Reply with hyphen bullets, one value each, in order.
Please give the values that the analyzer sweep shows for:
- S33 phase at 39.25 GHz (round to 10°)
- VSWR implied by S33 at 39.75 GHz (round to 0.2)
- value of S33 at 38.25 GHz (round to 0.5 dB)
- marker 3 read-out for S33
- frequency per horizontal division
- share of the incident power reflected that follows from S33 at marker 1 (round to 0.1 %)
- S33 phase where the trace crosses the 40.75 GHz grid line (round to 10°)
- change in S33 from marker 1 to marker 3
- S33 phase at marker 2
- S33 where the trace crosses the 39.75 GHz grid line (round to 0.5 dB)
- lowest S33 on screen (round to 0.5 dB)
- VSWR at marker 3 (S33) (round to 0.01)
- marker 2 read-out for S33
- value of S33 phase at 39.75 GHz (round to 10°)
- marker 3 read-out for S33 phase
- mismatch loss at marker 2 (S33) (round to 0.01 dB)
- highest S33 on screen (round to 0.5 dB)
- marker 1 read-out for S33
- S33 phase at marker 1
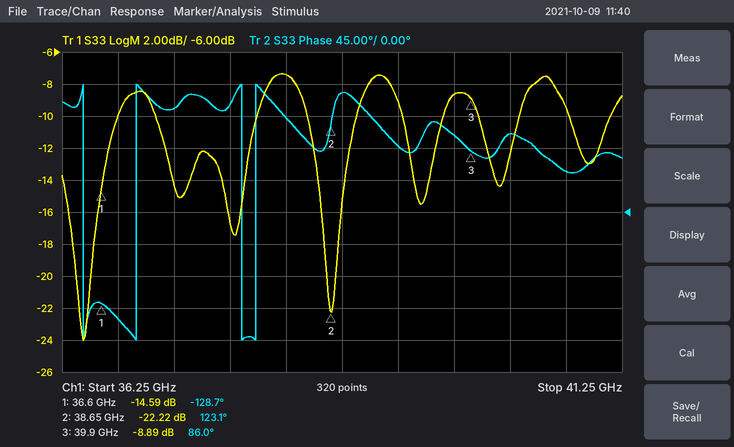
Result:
- 90°
- 2.2
- -7.5 dB
- -8.89 dB
- 500 MHz
- 3.5 %
- 60°
- 5.70 dB
- 123.1°
- -8.5 dB
- -24.0 dB
- 2.12
- -22.22 dB
- 110°
- 86.0°
- 0.03 dB
- -7.5 dB
- -14.59 dB
- -128.7°
